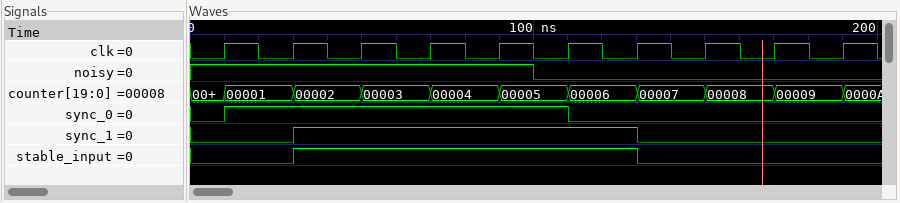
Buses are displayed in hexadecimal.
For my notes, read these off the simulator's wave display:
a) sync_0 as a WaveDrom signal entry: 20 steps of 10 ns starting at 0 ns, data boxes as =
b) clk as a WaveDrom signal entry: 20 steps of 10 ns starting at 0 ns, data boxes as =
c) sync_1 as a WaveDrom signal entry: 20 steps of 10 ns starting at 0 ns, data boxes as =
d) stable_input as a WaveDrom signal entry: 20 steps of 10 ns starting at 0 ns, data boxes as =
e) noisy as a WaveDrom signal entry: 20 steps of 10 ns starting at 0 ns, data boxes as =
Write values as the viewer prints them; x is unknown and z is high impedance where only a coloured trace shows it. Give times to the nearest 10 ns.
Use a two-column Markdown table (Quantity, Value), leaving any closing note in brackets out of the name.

| Quantity | Value |
|---|---|
| sync_0 as a WaveDrom signal entry: 20 steps of 10 ns starting at 0 ns, data boxes as = | {name: 'sync_0', wave: '01.........0........'} |
| clk as a WaveDrom signal entry: 20 steps of 10 ns starting at 0 ns, data boxes as = | {name: 'clk', wave: '01010101010101010101'} |
| sync_1 as a WaveDrom signal entry: 20 steps of 10 ns starting at 0 ns, data boxes as = | {name: 'sync_1', wave: '0..1.........0......'} |
| stable_input as a WaveDrom signal entry: 20 steps of 10 ns starting at 0 ns, data boxes as = | {name: 'stable_input', wave: '0..1.........0......'} |
| noisy as a WaveDrom signal entry: 20 steps of 10 ns starting at 0 ns, data boxes as = | {name: 'noisy', wave: '1.........0.........'} |
